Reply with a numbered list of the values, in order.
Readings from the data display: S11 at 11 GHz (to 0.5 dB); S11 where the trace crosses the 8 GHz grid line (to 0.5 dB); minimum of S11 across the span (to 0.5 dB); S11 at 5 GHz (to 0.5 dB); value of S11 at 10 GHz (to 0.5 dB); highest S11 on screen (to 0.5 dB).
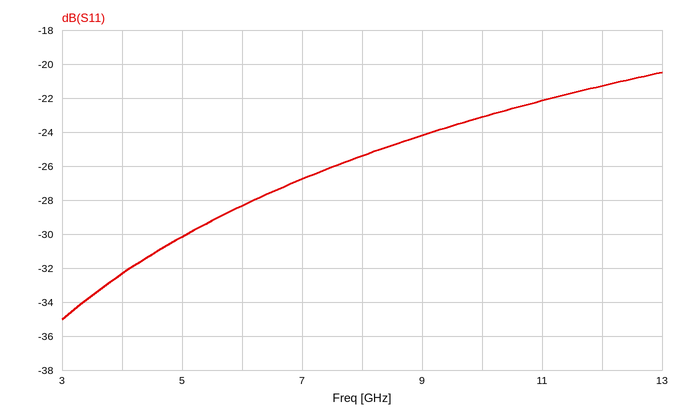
1. -22.0 dB
2. -25.5 dB
3. -35.0 dB
4. -30.0 dB
5. -23.0 dB
6. -20.5 dB
